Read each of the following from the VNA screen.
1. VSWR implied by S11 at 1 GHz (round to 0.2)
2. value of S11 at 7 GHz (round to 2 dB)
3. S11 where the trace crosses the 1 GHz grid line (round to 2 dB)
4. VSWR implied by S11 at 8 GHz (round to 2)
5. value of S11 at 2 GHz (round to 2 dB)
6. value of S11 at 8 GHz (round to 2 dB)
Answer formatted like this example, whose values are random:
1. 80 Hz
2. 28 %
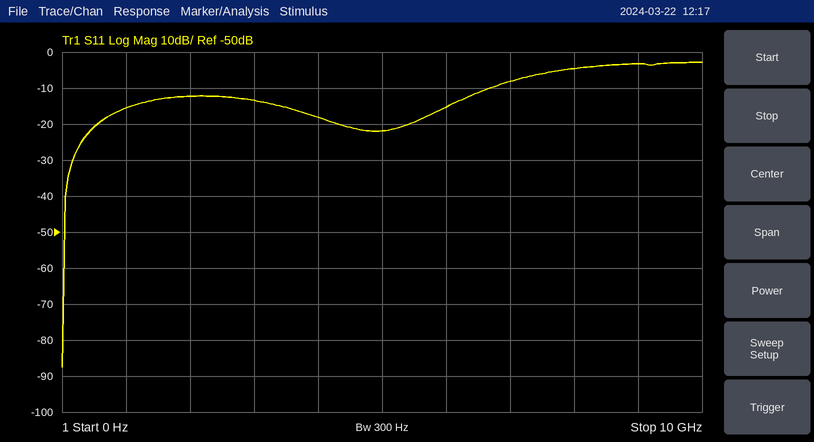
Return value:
1. 1.4
2. -8 dB
3. -16 dB
4. 4
5. -12 dB
6. -4 dB
